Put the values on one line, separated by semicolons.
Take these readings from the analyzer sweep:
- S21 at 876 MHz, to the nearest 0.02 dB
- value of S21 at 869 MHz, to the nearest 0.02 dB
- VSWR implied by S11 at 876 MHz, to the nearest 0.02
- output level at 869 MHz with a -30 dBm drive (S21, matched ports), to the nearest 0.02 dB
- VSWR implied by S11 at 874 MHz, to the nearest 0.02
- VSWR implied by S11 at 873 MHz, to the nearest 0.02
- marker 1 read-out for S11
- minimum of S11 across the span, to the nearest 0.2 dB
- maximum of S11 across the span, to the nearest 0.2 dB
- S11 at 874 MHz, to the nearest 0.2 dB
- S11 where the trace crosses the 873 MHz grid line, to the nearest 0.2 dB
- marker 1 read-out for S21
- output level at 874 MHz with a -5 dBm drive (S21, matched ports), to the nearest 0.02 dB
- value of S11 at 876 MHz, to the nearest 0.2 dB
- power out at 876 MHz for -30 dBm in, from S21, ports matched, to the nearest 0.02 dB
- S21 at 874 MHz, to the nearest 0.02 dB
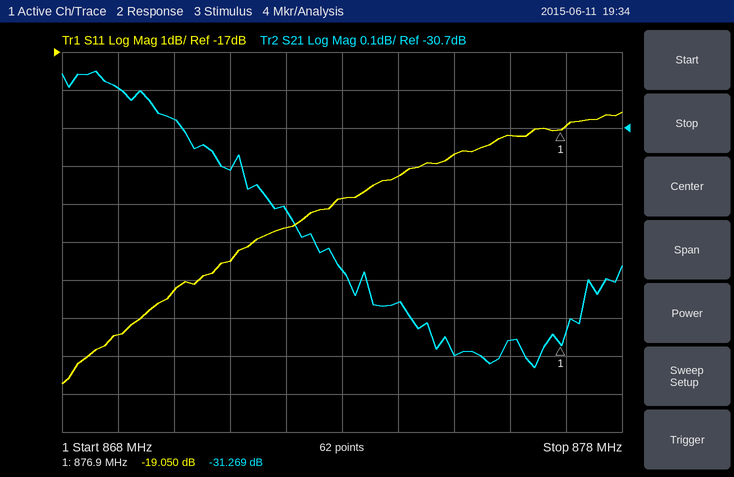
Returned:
-31.26 dB; -30.60 dB; 1.24; -60.60 dBm; 1.22; 1.20; -19.050 dB; -25.8 dB; -18.6 dB; -20.2 dB; -20.8 dB; -31.269 dB; -36.16 dBm; -19.2 dB; -61.26 dBm; -31.16 dB
